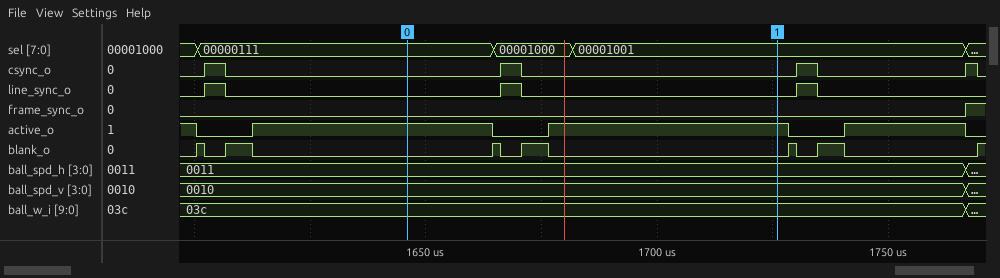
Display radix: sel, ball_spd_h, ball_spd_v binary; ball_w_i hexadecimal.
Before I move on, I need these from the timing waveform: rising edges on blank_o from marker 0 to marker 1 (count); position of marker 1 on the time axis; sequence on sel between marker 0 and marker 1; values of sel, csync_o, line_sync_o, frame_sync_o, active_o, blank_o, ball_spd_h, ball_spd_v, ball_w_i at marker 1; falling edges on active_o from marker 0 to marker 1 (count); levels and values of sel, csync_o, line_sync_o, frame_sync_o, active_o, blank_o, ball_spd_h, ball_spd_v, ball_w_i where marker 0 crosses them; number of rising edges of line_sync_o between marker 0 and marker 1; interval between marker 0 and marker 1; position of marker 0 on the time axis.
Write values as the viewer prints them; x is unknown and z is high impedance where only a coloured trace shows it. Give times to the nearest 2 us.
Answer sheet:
2
1726 us
00000111, 00001000, 00001001
sel=00001001, csync_o=0, line_sync_o=0, frame_sync_o=0, active_o=1, blank_o=0, ball_spd_h=0011, ball_spd_v=0010, ball_w_i=03c
1
sel=00000111, csync_o=0, line_sync_o=0, frame_sync_o=0, active_o=1, blank_o=0, ball_spd_h=0011, ball_spd_v=0010, ball_w_i=03c
1
80 us
1646 us
